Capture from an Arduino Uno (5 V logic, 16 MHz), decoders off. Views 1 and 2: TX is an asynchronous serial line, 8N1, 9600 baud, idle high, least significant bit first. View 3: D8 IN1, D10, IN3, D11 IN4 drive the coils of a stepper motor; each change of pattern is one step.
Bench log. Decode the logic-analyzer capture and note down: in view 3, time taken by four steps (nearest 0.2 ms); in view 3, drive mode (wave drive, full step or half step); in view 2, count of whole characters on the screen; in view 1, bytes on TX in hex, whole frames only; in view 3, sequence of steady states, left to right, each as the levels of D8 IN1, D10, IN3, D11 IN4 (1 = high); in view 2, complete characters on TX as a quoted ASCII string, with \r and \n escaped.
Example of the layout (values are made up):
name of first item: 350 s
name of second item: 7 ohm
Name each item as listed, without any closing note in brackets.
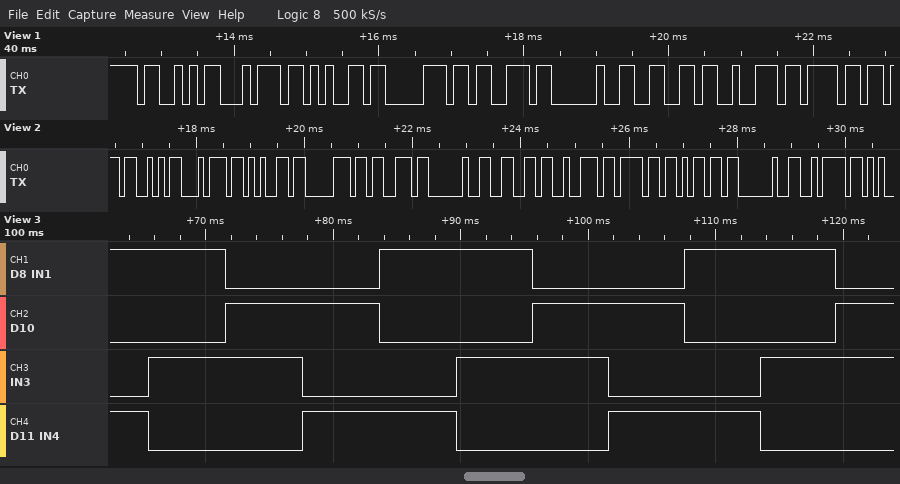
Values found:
in view 3, time taken by four steps: 24.2 ms
in view 3, drive mode: full step
in view 2, count of whole characters on the screen: 12
in view 1, bytes on TX in hex, whole frames only: 53 74 65 70 73 20 66 72 6F
in view 3, sequence of steady states, left to right, each as the levels of D8 IN1, D10, IN3, D11 IN4: 1001 1010 0110 0101 1001 1010 0110 0101 1001 1010 0110
in view 2, complete characters on TX as a quoted ASCII string, with \r and \n escaped: "Steps from z"
